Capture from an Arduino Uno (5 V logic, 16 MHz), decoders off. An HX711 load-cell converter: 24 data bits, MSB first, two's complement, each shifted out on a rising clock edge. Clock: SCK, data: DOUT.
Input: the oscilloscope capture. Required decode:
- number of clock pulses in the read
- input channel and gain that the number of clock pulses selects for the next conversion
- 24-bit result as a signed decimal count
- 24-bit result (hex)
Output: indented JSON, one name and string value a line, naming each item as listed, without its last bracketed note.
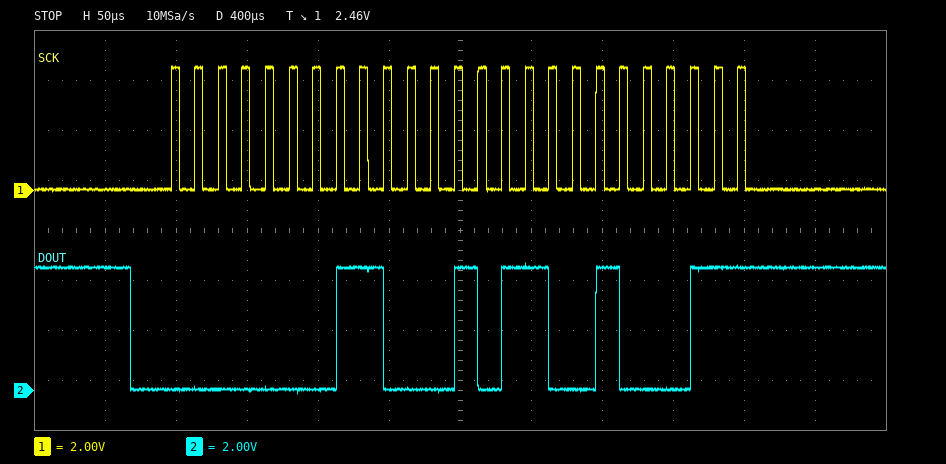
{
  "number of clock pulses in the read": "25",
  "input channel and gain that the number of clock pulses selects for the next conversion": "channel A, gain 128",
  "24-bit result as a signed decimal count": "101155",
  "24-bit result": "0x018B23"
}
